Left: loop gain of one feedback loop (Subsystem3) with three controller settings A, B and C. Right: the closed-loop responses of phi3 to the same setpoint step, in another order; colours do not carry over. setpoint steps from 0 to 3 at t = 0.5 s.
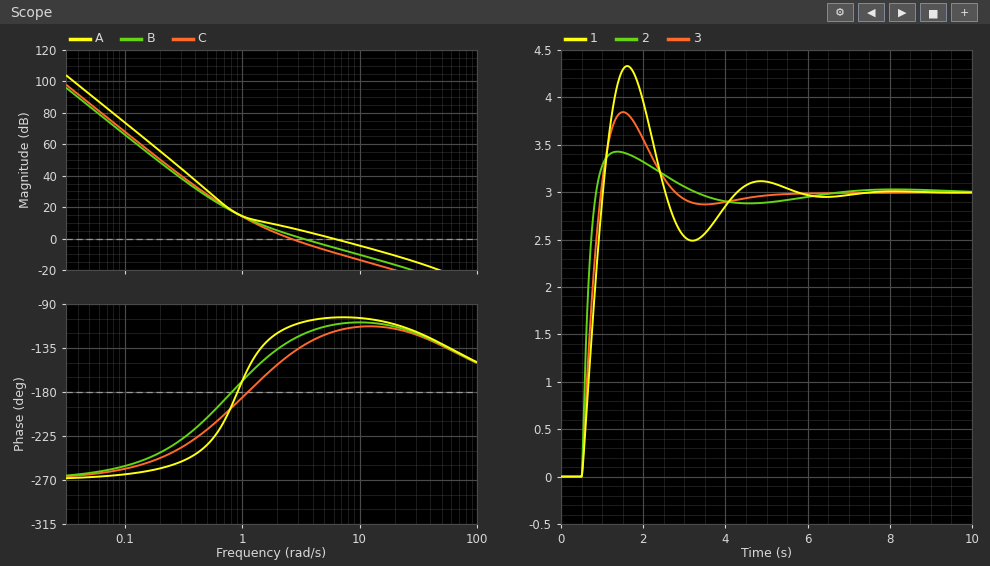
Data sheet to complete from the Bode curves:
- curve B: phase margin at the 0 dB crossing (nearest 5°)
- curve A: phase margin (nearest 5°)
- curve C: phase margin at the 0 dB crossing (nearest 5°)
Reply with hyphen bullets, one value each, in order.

- 60°
- 75°
- 40°
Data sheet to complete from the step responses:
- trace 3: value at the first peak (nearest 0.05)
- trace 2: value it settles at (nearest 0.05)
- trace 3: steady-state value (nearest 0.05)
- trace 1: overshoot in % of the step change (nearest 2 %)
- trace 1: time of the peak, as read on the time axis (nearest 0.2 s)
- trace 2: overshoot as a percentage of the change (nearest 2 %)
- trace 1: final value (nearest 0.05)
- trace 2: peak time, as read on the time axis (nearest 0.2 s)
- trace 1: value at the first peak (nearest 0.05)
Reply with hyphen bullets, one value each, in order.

- 3.85
- 3.00
- 3.00
- 44 %
- 1.6 s
- 14 %
- 3.00
- 1.4 s
- 4.35
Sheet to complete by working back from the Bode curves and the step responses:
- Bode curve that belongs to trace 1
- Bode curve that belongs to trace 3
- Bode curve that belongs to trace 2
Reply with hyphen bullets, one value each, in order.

- C
- B
- A
